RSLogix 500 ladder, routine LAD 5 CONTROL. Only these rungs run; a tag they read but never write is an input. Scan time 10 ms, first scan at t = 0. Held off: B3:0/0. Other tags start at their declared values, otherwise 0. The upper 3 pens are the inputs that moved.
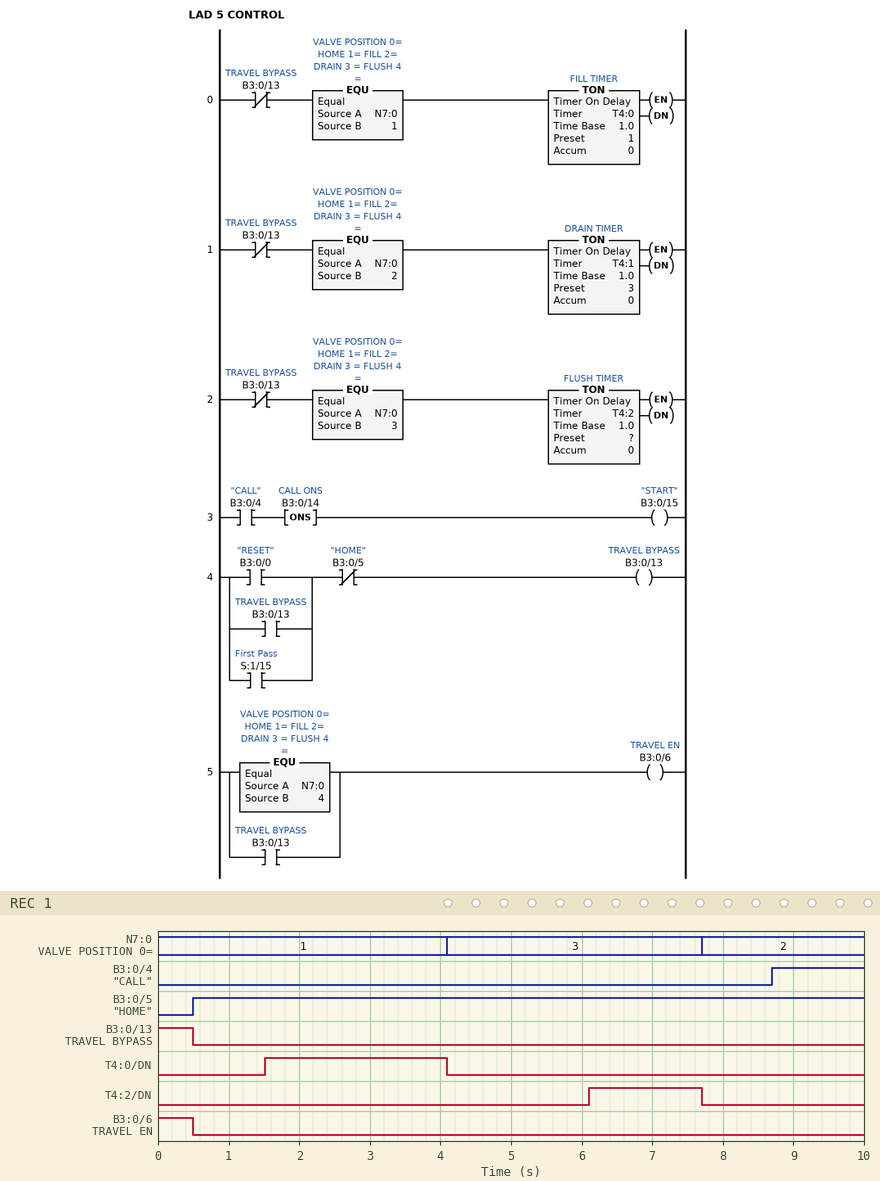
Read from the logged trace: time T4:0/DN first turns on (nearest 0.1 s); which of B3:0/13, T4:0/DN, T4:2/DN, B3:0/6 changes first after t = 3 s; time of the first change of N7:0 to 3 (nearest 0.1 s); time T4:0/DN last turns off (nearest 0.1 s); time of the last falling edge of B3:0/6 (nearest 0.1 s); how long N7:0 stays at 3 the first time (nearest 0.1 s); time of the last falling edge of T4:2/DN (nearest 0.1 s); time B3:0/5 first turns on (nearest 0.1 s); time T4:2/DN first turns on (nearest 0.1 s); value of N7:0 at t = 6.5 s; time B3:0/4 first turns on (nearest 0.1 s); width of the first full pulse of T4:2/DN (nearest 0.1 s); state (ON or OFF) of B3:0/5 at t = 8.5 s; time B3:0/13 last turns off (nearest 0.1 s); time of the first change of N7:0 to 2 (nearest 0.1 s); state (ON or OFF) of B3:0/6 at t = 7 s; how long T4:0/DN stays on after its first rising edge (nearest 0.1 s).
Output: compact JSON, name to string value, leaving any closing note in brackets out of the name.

{"time T4:0/DN first turns on": "1.5 s", "which of B3:0/13, T4:0/DN, T4:2/DN, B3:0/6 changes first after t = 3 s": "T4:0/DN", "time of the first change of N7:0 to 3": "4.1 s", "time T4:0/DN last turns off": "4.1 s", "time of the last falling edge of B3:0/6": "0.5 s", "how long N7:0 stays at 3 the first time": "3.6 s", "time of the last falling edge of T4:2/DN": "7.7 s", "time B3:0/5 first turns on": "0.5 s", "time T4:2/DN first turns on": "6.1 s", "value of N7:0 at t = 6.5 s": "3", "time B3:0/4 first turns on": "8.7 s", "width of the first full pulse of T4:2/DN": "1.6 s", "state (ON or OFF) of B3:0/5 at t = 8.5 s": "ON", "time B3:0/13 last turns off": "0.5 s", "time of the first change of N7:0 to 2": "7.7 s", "state (ON or OFF) of B3:0/6 at t = 7 s": "OFF", "how long T4:0/DN stays on after its first rising edge": "2.6 s"}
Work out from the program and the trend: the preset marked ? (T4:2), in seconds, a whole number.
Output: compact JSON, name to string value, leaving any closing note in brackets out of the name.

{"the preset marked ? (T4:2), in seconds, a whole number": "2 s"}
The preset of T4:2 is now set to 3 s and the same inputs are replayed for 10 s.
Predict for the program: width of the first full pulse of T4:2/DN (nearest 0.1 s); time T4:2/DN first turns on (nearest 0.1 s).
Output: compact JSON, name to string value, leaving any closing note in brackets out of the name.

{"width of the first full pulse of T4:2/DN": "0.6 s", "time T4:2/DN first turns on": "7.1 s"}
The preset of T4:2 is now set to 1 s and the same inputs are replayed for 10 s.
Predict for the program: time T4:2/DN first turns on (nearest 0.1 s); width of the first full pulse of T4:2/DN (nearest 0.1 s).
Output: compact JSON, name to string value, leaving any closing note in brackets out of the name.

{"time T4:2/DN first turns on": "5.1 s", "width of the first full pulse of T4:2/DN": "2.6 s"}
